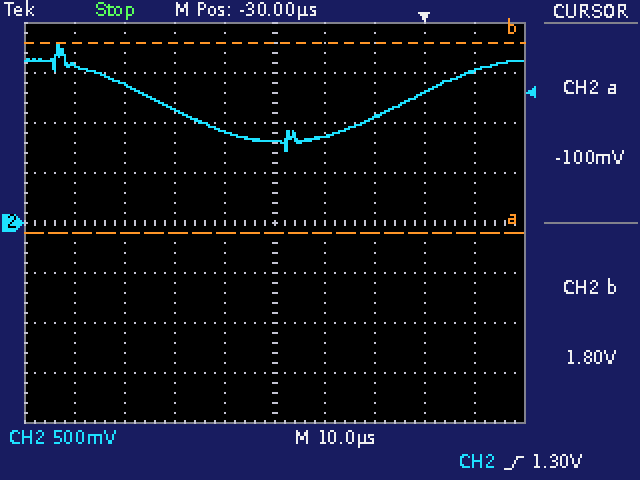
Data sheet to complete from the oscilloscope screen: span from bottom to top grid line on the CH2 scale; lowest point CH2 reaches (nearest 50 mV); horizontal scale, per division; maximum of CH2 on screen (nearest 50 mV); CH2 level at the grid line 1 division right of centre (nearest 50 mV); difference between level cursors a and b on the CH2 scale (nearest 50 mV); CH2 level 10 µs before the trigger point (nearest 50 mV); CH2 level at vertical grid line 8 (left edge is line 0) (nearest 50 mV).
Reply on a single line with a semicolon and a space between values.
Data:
4 V; 700 mV; 10 µs; 1.80 V; 850 mV; 1.90 V; 1.05 V; 1.30 V
